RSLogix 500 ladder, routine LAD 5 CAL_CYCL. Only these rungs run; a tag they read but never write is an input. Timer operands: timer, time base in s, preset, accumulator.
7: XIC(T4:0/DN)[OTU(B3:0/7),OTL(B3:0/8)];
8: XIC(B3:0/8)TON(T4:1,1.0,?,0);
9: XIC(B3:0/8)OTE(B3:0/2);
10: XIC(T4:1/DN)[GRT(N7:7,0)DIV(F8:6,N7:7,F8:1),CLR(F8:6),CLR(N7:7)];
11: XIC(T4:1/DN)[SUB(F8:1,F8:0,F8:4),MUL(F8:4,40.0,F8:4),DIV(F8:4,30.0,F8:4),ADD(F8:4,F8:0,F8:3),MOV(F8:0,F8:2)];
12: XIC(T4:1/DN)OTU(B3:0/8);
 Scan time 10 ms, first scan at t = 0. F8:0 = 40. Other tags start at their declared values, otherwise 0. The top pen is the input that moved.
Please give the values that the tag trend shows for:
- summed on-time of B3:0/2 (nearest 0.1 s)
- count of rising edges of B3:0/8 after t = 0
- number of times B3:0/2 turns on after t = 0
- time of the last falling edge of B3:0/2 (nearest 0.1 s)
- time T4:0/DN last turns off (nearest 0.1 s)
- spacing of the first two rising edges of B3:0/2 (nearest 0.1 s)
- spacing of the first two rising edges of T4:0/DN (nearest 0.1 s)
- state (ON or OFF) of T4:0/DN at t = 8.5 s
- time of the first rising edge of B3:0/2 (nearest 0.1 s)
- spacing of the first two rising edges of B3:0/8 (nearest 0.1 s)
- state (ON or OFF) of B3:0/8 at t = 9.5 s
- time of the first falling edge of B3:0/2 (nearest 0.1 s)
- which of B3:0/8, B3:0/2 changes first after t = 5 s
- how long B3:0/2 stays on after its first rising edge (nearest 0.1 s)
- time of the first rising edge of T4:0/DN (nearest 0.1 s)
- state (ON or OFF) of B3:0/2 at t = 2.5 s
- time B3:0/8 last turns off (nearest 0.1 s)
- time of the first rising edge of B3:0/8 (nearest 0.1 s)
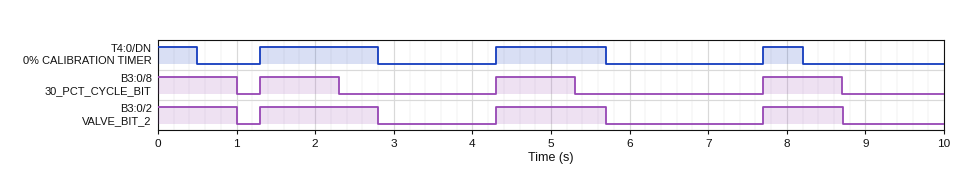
4.9 s
3
3
8.7 s
8.2 s
3.0 s
3.0 s
OFF
1.3 s
3.0 s
OFF
1.0 s
B3:0/8
1.5 s
1.3 s
ON
8.7 s
1.3 s
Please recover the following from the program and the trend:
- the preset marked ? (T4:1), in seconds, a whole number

1 s
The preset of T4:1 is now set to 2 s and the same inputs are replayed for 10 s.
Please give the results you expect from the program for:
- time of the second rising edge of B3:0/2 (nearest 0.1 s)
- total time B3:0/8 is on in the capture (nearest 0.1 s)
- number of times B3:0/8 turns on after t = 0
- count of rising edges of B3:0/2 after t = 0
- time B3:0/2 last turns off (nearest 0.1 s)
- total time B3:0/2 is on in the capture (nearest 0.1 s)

7.7 s
6.0 s
2
2
9.7 s
6.8 s
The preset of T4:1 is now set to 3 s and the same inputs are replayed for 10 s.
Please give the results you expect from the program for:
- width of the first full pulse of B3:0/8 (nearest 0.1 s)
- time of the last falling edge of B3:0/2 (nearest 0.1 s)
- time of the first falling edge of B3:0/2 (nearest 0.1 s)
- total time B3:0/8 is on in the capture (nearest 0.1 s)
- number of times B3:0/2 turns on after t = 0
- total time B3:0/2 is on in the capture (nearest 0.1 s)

3.0 s
7.3 s
3.0 s
8.3 s
2
8.3 s
